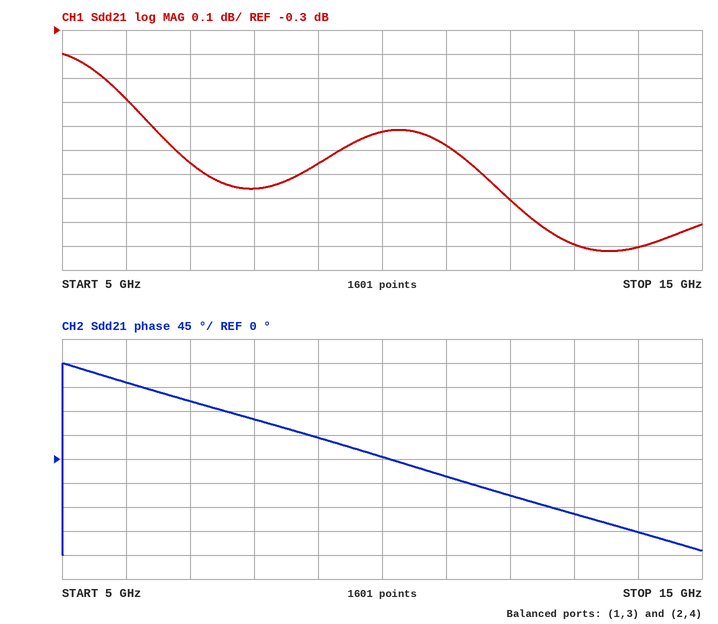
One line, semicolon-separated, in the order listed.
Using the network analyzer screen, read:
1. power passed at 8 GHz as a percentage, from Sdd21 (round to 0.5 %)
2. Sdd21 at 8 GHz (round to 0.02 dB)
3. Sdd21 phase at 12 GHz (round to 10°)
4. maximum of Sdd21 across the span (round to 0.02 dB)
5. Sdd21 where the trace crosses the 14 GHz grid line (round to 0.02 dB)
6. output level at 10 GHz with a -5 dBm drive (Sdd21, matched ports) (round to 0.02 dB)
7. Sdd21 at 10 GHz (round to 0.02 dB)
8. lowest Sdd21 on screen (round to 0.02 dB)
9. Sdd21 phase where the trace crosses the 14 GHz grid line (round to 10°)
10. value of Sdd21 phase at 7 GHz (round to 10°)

80.0 %; -0.96 dB; -70°; -0.40 dB; -1.20 dB; -5.72 dBm; -0.72 dB; -1.22 dB; -140°; 110°
